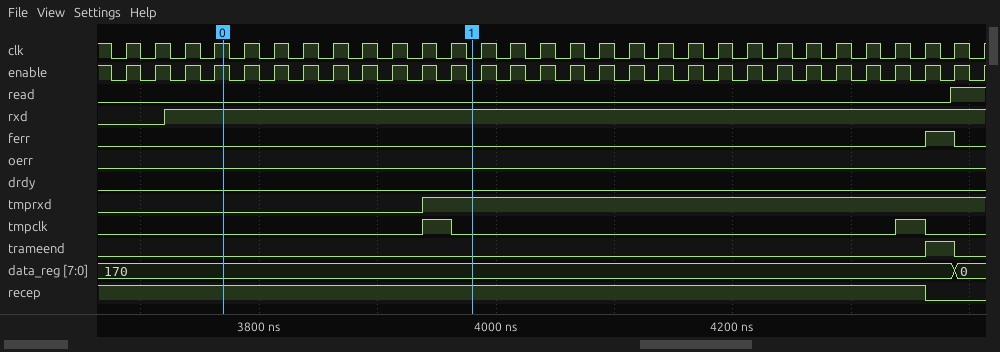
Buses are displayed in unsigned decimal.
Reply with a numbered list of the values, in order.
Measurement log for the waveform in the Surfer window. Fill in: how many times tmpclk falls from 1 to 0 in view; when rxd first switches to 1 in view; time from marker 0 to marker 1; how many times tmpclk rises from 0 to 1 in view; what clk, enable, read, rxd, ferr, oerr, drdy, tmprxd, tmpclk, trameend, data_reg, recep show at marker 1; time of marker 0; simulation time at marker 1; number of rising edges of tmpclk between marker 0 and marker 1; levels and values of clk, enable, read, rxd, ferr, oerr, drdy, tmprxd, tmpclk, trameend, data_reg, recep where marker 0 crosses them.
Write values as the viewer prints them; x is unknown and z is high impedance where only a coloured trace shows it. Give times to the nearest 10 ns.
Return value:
1. 2
2. 3720 ns
3. 210 ns
4. 2
5. clk=0, enable=0, read=0, rxd=1, ferr=0, oerr=0, drdy=0, tmprxd=1, tmpclk=0, trameend=0, data_reg=170, recep=1
6. 3770 ns
7. 3980 ns
8. 1
9. clk=1, enable=1, read=0, rxd=1, ferr=0, oerr=0, drdy=0, tmprxd=0, tmpclk=0, trameend=0, data_reg=170, recep=1
